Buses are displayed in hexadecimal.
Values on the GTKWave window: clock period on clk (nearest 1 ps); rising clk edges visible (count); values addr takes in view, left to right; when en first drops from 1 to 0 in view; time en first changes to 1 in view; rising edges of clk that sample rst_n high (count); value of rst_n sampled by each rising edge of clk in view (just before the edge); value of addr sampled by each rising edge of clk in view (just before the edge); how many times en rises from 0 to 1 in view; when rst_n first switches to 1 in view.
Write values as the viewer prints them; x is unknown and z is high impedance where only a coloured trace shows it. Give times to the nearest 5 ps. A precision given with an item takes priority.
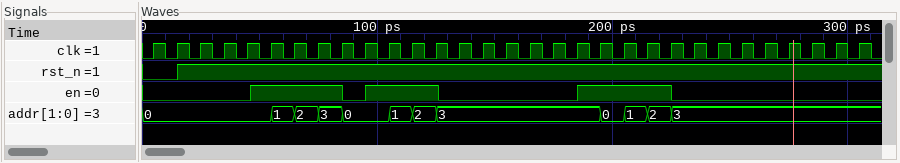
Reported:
10 ps
31
0, 1, 2, 3, 0, 1, 2, 3, 0, 1, 2, 3
85 ps
45 ps
29
0 0 1 1 1 1 1 1 1 1 1 1 1 1 1 1 1 1 1 1 1 1 1 1 1 1 1 1 1 1 1
0, 0, 0, 0, 0, 0, 1, 2, 3, 0, 0, 1, 2, 3, 3, 3, 3, 3, 3, 3, 0, 1, 2, 3, 3, 3, 3, 3, 3, 3, 3
3
15 ps
